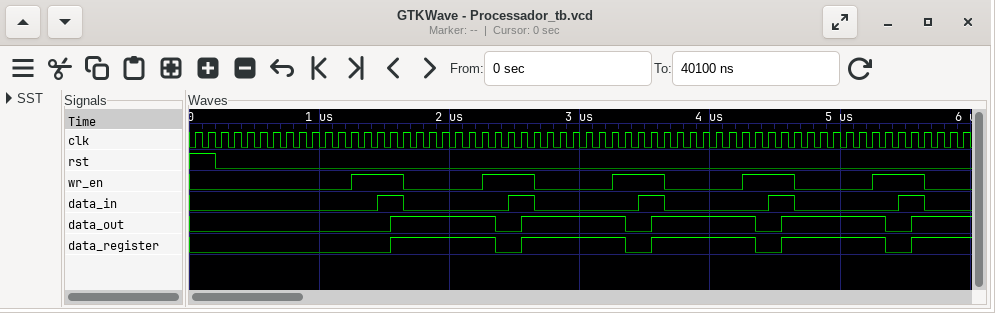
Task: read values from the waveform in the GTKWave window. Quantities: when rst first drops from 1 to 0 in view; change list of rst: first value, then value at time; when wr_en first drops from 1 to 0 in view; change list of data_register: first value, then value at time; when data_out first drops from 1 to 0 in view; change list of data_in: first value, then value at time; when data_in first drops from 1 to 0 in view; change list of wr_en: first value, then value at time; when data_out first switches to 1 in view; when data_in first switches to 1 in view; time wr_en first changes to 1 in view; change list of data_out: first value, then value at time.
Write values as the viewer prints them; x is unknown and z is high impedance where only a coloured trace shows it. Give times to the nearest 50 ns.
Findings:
200 ns
1, 0 at 200 ns
1650 ns
0, 1 at 1550 ns, 0 at 2350 ns, 1 at 2550 ns, 0 at 3350 ns, 1 at 3550 ns, 0 at 4350 ns, 1 at 4550 ns, 0 at 5350 ns, 1 at 5550 ns
2350 ns
0, 1 at 1450 ns, 0 at 1650 ns, 1 at 2450 ns, 0 at 2650 ns, 1 at 3450 ns, 0 at 3650 ns, 1 at 4450 ns, 0 at 4650 ns, 1 at 5450 ns, 0 at 5650 ns
1650 ns
0, 1 at 1250 ns, 0 at 1650 ns, 1 at 2250 ns, 0 at 2650 ns, 1 at 3250 ns, 0 at 3650 ns, 1 at 4250 ns, 0 at 4650 ns, 1 at 5250 ns, 0 at 5650 ns
1550 ns
1450 ns
1250 ns
0, 1 at 1550 ns, 0 at 2350 ns, 1 at 2550 ns, 0 at 3350 ns, 1 at 3550 ns, 0 at 4350 ns, 1 at 4550 ns, 0 at 5350 ns, 1 at 5550 ns
